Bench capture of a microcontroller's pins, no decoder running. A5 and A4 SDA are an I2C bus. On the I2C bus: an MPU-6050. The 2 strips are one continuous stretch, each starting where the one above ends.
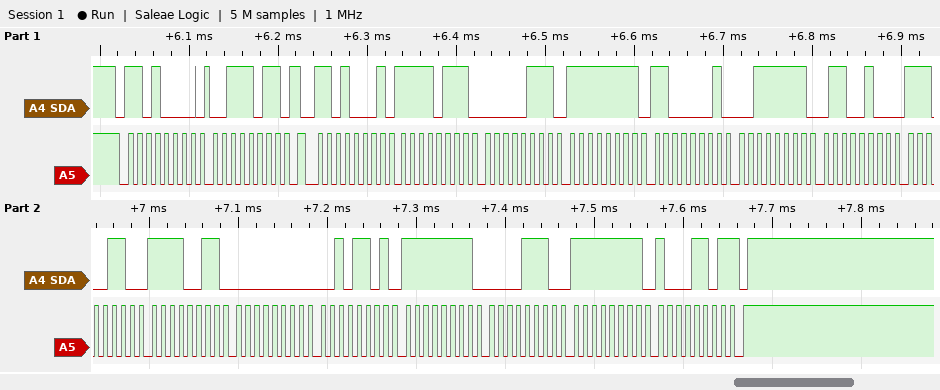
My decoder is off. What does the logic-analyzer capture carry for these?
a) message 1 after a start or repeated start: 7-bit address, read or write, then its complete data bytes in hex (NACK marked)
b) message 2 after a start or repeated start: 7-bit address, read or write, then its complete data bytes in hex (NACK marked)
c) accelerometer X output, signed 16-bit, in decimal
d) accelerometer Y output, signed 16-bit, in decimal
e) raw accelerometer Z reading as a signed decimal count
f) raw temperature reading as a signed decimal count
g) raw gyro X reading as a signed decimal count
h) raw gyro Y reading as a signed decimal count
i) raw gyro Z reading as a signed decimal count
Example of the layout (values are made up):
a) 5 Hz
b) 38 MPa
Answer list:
a) 0x68 write: 3B
b) 0x68 read: F7 07 FF C1 3F 64 E6 F3 00 2D FF 0E FF 8D NACK
c) -2297
d) -63
e) 16228
f) -6413
g) 45
h) -242
i) -115
